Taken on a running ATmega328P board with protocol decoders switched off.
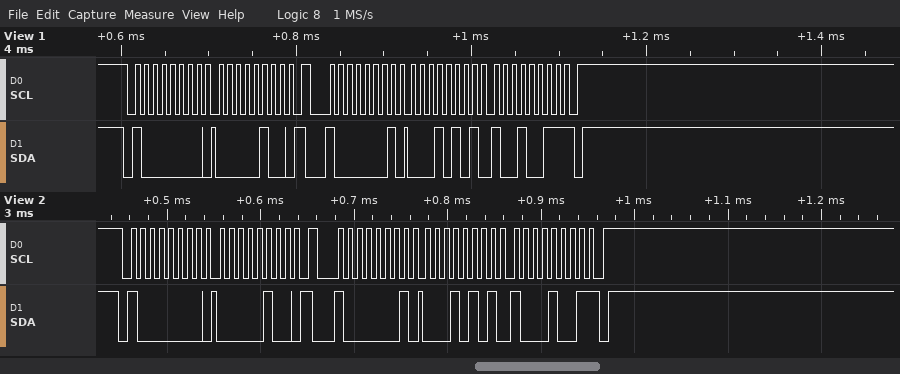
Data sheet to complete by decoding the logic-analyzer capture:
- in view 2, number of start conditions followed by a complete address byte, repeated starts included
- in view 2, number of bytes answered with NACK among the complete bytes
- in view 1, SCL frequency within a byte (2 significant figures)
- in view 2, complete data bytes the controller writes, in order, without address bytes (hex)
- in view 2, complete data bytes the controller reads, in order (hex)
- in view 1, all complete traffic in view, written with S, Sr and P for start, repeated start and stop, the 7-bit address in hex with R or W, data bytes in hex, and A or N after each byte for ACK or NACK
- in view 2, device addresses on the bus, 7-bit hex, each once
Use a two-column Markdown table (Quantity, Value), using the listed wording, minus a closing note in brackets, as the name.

| Quantity | Value |
|---|---|
| in view 2, number of start conditions followed by a complete address byte, repeated starts included | 2 |
| in view 2, number of bytes answered with NACK among the complete bytes | 1 |
| in view 1, SCL frequency within a byte | 100 kHz |
| in view 2, complete data bytes the controller writes, in order, without address bytes | 04 |
| in view 2, complete data bytes the controller reads, in order | 15 89 |
| in view 1, all complete traffic in view, written with S, Sr and P for start, repeated start and stop, the 7-bit address in hex with R or W, data bytes in hex, and A or N after each byte for ACK or NACK | S 40W A 04 A Sr 40R A 15 A 93 N P |
| in view 2, device addresses on the bus, 7-bit hex, each once | 0x40 |
